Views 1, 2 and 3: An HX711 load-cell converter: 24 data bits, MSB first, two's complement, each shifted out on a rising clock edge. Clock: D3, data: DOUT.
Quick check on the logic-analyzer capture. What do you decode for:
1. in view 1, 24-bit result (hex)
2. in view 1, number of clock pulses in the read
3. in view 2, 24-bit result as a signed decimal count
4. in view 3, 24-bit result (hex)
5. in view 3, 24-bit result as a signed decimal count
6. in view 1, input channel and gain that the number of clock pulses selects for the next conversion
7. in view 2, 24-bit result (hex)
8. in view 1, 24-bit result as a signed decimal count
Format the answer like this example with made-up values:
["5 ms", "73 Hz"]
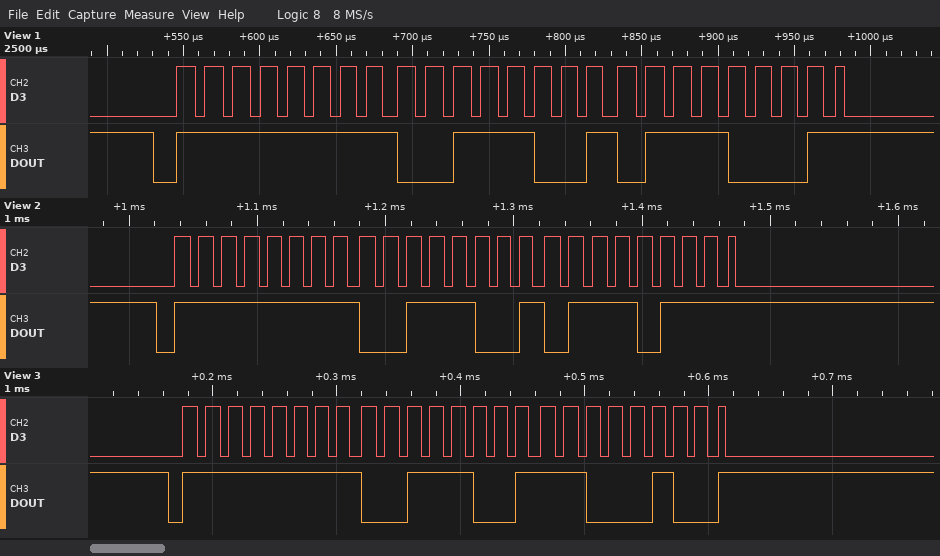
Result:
["0xFF3971", "25", "-50825", "0xFF39C4", "-50748", "channel A, gain 128", "0xFF3977", "-50831"]
